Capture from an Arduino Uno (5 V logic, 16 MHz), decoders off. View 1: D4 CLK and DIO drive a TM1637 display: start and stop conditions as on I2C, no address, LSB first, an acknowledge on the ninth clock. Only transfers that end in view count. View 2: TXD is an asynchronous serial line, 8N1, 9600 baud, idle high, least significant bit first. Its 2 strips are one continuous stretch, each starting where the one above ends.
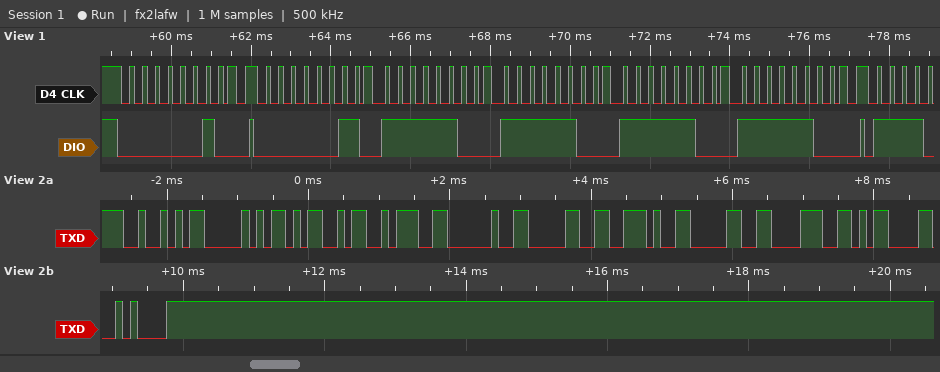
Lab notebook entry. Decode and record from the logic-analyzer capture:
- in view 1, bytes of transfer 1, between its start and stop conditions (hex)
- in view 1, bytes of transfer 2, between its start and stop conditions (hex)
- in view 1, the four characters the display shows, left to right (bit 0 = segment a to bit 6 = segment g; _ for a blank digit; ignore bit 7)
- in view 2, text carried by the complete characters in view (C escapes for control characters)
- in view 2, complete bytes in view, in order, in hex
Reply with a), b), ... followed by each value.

a) 40
b) C0 3F 3F 3F 3F
c) 0000
d) "RPM: 0.08\r\n"
e) 0x52 0x50 0x4D 0x3A 0x20 0x30 0x2E 0x30 0x38 0x0D 0x0A
